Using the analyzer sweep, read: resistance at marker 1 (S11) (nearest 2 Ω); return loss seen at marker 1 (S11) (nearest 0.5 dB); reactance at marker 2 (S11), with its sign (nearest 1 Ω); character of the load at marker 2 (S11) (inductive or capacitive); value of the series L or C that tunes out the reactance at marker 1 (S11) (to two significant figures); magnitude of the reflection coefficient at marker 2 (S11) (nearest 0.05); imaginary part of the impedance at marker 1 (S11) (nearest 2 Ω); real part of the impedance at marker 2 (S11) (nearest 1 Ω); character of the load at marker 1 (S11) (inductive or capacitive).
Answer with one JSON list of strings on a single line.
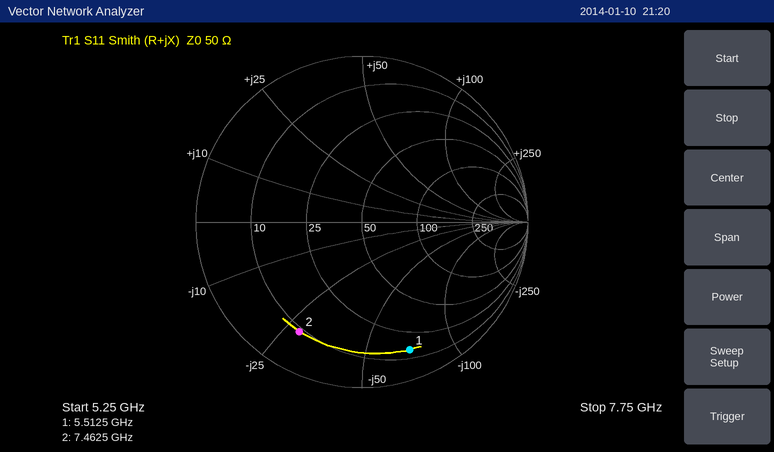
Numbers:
["14 Ω", "1.5 dB", "-28 Ω", "capacitive", "2.0 nH", "0.75", "-70 Ω", "9 Ω", "capacitive"]
